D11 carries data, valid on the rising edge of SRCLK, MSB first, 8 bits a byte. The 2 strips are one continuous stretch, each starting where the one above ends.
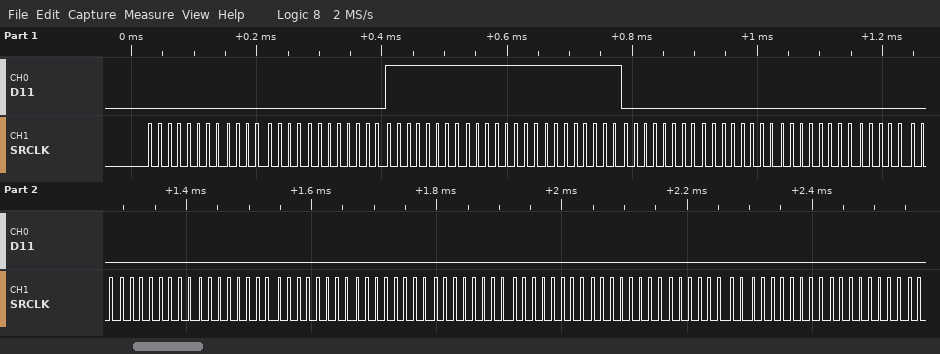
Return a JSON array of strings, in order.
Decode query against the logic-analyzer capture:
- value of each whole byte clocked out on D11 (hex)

["0x00 0x00 0x00 0xFF 0xFF 0xFF 0x00 0x00 0x00 0x00 0x00 0x00 0x00 0x00 0x00 0x00 0x00 0x00 0x00 0x00"]
